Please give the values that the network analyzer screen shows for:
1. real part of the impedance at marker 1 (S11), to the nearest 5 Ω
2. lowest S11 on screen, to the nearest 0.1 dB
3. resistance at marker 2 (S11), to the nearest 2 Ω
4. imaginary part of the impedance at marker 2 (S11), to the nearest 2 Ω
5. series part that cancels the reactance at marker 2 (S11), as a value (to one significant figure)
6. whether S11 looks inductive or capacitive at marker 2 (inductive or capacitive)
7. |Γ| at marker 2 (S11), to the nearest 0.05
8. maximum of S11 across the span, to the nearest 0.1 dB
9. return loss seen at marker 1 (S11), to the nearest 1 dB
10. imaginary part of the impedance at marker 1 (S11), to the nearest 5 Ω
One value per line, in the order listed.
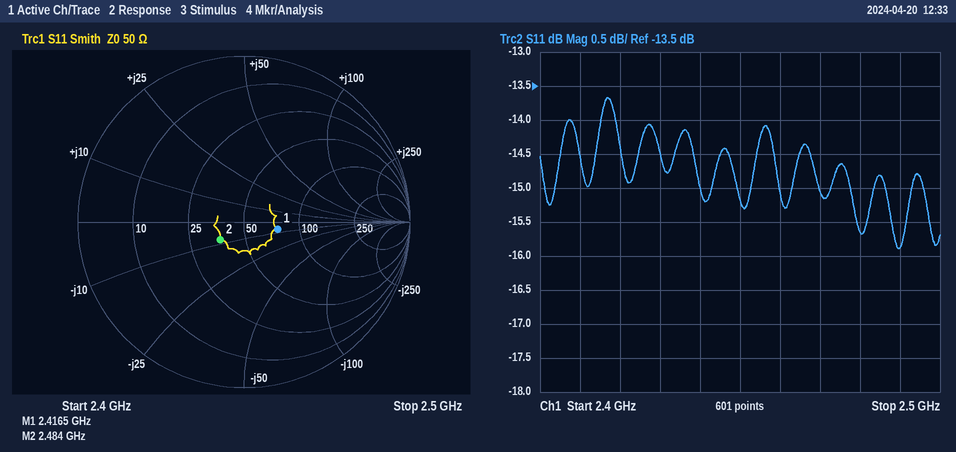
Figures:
75 Ω
-15.9 dB
36 Ω
-8 Ω
500 pH
capacitive
0.20
-13.7 dB
14 dB
-5 Ω
